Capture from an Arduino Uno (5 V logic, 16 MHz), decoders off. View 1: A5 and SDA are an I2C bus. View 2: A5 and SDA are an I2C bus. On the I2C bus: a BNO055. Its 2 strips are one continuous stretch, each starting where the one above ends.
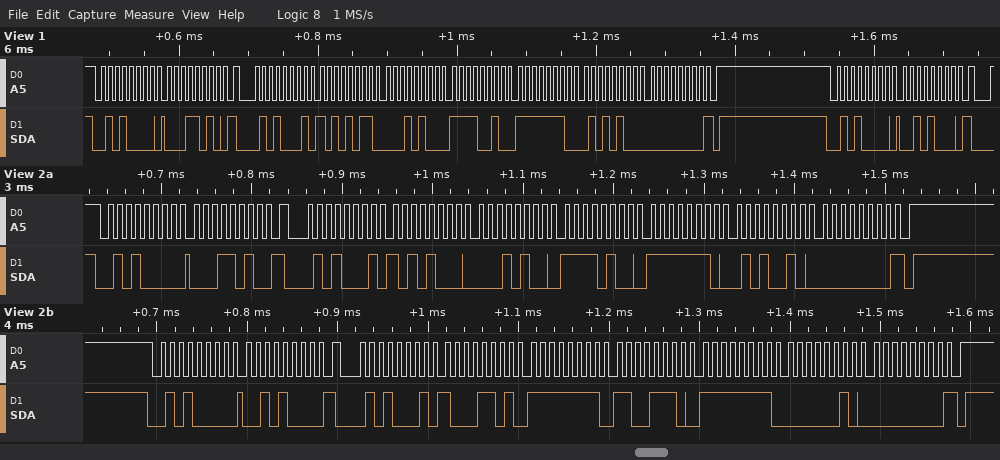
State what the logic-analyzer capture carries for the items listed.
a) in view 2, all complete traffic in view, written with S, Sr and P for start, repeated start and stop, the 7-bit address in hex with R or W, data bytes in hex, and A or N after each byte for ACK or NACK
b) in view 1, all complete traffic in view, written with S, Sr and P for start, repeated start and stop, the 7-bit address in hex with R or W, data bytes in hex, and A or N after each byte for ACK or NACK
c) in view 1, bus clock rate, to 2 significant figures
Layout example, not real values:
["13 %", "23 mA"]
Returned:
["S 28W A 1A A Sr 28R A A8 A 14 A F4 A FE A 52 A 00 N P S 28W A 28 A Sr 28R A 8D A FF A CE A FF A 02 A 00 N P", "S 28W A 1A A Sr 28R A AB A 14 A F2 A FE A 54 A 00 N P S 28W A 28 A", "100 kHz"]
